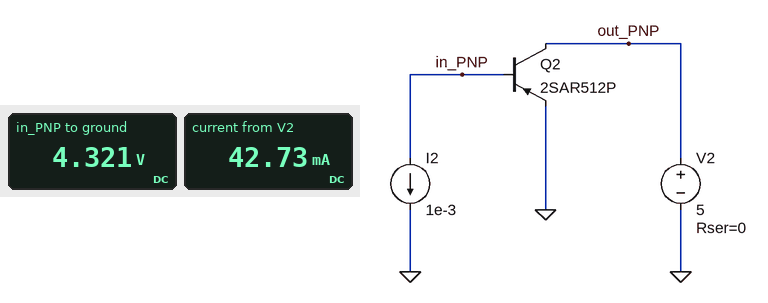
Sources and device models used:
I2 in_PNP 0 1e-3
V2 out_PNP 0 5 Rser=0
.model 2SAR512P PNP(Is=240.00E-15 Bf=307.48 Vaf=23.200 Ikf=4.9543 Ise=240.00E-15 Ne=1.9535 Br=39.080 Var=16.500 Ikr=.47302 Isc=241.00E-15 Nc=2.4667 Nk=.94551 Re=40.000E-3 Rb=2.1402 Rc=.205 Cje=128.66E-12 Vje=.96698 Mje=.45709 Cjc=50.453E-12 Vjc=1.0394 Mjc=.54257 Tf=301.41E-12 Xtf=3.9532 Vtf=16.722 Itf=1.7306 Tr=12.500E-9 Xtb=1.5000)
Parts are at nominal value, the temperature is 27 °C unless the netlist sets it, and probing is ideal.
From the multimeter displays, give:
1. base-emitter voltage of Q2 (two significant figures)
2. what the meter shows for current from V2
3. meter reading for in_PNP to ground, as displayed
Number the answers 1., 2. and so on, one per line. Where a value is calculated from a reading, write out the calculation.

1. 4.321 V = 4.3 V
2. 42.73 mA
3. 4.321 V
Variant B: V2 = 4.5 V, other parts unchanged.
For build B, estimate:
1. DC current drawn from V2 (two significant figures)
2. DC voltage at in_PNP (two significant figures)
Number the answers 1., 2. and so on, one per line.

1. 42 mA
2. 3.8 V
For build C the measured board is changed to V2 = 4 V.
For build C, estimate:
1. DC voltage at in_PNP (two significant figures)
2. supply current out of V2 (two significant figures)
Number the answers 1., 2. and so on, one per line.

1. 3.3 V
2. 41 mA
